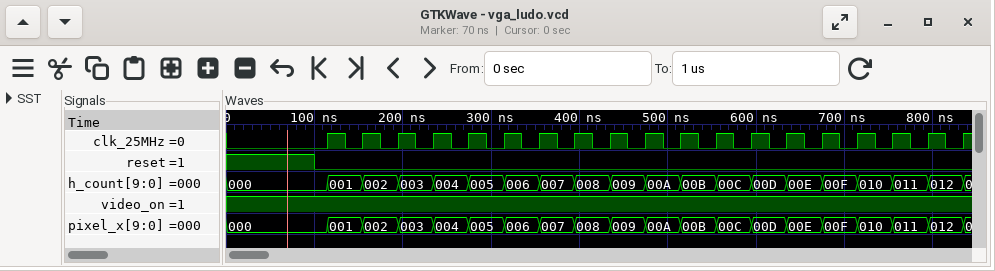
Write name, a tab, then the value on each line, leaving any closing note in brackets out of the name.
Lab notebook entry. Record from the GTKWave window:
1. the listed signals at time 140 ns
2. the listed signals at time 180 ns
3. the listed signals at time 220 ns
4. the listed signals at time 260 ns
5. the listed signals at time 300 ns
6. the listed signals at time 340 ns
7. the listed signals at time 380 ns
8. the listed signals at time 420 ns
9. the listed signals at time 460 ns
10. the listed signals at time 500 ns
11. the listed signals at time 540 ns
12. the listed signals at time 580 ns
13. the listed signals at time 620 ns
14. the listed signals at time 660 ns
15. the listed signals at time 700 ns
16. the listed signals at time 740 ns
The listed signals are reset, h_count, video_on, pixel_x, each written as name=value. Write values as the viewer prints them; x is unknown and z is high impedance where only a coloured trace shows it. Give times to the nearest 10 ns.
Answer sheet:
the listed signals at time 140 ns	reset=0, h_count=001, video_on=1, pixel_x=001
the listed signals at time 180 ns	reset=0, h_count=002, video_on=1, pixel_x=002
the listed signals at time 220 ns	reset=0, h_count=003, video_on=1, pixel_x=003
the listed signals at time 260 ns	reset=0, h_count=004, video_on=1, pixel_x=004
the listed signals at time 300 ns	reset=0, h_count=005, video_on=1, pixel_x=005
the listed signals at time 340 ns	reset=0, h_count=006, video_on=1, pixel_x=006
the listed signals at time 380 ns	reset=0, h_count=007, video_on=1, pixel_x=007
the listed signals at time 420 ns	reset=0, h_count=008, video_on=1, pixel_x=008
the listed signals at time 460 ns	reset=0, h_count=009, video_on=1, pixel_x=009
the listed signals at time 500 ns	reset=0, h_count=00A, video_on=1, pixel_x=00A
the listed signals at time 540 ns	reset=0, h_count=00B, video_on=1, pixel_x=00B
the listed signals at time 580 ns	reset=0, h_count=00C, video_on=1, pixel_x=00C
the listed signals at time 620 ns	reset=0, h_count=00D, video_on=1, pixel_x=00D
the listed signals at time 660 ns	reset=0, h_count=00E, video_on=1, pixel_x=00E
the listed signals at time 700 ns	reset=0, h_count=00F, video_on=1, pixel_x=00F
the listed signals at time 740 ns	reset=0, h_count=010, video_on=1, pixel_x=010
